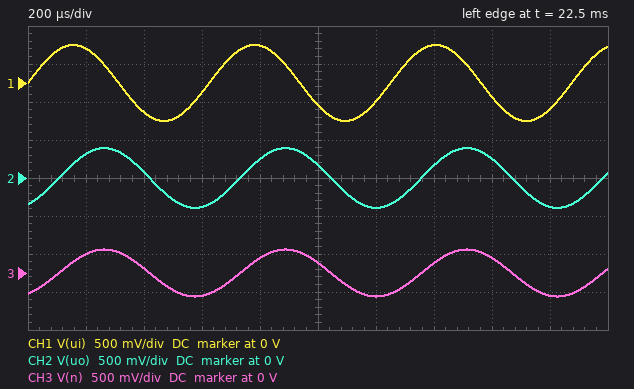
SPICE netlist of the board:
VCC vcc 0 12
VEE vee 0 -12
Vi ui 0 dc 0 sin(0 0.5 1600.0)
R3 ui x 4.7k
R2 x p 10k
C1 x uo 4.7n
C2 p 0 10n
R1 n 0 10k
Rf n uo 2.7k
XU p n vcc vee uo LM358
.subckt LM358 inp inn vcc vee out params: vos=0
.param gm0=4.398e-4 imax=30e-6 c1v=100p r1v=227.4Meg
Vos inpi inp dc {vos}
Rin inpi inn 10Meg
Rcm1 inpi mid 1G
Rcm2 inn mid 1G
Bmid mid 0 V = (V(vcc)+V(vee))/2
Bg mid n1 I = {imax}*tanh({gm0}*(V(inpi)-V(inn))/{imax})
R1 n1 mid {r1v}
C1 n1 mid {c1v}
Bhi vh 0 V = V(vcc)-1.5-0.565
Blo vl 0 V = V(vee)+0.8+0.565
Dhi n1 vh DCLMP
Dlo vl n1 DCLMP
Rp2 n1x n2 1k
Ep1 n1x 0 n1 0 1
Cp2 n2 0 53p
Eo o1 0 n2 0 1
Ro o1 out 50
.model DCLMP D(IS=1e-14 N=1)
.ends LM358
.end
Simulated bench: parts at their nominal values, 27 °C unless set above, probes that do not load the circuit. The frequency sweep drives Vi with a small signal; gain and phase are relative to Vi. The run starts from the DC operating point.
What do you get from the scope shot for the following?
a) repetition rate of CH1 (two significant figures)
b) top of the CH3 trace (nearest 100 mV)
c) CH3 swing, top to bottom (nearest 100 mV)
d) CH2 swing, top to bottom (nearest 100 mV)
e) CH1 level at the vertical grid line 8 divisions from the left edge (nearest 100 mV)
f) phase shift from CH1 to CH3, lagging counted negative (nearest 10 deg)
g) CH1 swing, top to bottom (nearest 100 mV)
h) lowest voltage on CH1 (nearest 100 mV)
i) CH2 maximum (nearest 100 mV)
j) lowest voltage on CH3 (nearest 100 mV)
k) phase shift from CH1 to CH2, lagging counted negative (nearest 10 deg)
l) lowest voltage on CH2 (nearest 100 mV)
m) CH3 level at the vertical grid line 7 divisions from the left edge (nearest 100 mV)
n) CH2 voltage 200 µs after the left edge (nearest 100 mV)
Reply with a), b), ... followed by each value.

a) 1.6 kHz
b) 300 mV
c) 600 mV
d) 800 mV
e) -200 mV
f) -60 deg
g) 1.0 V
h) -500 mV
i) 400 mV
j) -300 mV
k) -60 deg
l) -400 mV
m) 100 mV
n) 300 mV
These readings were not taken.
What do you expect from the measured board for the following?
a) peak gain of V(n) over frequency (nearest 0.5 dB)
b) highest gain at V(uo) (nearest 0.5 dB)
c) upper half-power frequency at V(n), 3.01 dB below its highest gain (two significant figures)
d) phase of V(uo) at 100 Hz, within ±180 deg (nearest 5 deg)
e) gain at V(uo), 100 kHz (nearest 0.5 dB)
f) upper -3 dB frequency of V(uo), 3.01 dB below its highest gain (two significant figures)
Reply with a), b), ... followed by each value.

a) 0 dB
b) 2.0 dB
c) 1.3 kHz
d) -5 deg
e) -52.5 dB
f) 1.3 kHz
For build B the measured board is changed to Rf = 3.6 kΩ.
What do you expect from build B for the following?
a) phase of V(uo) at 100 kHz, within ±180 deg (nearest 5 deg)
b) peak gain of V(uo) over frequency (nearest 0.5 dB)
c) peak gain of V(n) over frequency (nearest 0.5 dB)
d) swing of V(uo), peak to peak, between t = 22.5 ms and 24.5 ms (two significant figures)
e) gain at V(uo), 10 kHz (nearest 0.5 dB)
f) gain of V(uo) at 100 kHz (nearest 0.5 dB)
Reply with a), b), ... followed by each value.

a) 120 deg
b) 2.5 dB
c) 0 dB
d) 850 mV
e) -18.5 dB
f) -52.0 dB
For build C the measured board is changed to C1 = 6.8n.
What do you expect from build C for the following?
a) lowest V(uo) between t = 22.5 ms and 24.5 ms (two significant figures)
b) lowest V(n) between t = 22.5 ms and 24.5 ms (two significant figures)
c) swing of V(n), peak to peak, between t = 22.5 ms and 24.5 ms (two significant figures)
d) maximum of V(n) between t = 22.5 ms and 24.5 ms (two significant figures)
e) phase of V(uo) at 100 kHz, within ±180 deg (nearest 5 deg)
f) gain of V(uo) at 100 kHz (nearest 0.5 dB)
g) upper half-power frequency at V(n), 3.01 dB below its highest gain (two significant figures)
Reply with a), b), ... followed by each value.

a) -410 mV
b) -320 mV
c) 650 mV
d) 320 mV
e) 110 deg
f) -53.5 dB
g) 1.4 kHz
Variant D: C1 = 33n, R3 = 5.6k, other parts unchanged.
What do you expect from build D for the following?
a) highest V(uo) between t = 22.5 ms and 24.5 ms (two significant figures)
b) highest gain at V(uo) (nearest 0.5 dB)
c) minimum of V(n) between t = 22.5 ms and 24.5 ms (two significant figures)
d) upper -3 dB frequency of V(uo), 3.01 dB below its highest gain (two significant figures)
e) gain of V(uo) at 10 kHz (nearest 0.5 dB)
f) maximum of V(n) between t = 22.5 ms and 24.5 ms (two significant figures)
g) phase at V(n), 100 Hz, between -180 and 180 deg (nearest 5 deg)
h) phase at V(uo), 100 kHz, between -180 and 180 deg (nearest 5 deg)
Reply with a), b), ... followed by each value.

a) 460 mV
b) 5.0 dB
c) -360 mV
d) 1.4 kHz
e) -35.0 dB
f) 360 mV
g) -5 deg
h) 85 deg
